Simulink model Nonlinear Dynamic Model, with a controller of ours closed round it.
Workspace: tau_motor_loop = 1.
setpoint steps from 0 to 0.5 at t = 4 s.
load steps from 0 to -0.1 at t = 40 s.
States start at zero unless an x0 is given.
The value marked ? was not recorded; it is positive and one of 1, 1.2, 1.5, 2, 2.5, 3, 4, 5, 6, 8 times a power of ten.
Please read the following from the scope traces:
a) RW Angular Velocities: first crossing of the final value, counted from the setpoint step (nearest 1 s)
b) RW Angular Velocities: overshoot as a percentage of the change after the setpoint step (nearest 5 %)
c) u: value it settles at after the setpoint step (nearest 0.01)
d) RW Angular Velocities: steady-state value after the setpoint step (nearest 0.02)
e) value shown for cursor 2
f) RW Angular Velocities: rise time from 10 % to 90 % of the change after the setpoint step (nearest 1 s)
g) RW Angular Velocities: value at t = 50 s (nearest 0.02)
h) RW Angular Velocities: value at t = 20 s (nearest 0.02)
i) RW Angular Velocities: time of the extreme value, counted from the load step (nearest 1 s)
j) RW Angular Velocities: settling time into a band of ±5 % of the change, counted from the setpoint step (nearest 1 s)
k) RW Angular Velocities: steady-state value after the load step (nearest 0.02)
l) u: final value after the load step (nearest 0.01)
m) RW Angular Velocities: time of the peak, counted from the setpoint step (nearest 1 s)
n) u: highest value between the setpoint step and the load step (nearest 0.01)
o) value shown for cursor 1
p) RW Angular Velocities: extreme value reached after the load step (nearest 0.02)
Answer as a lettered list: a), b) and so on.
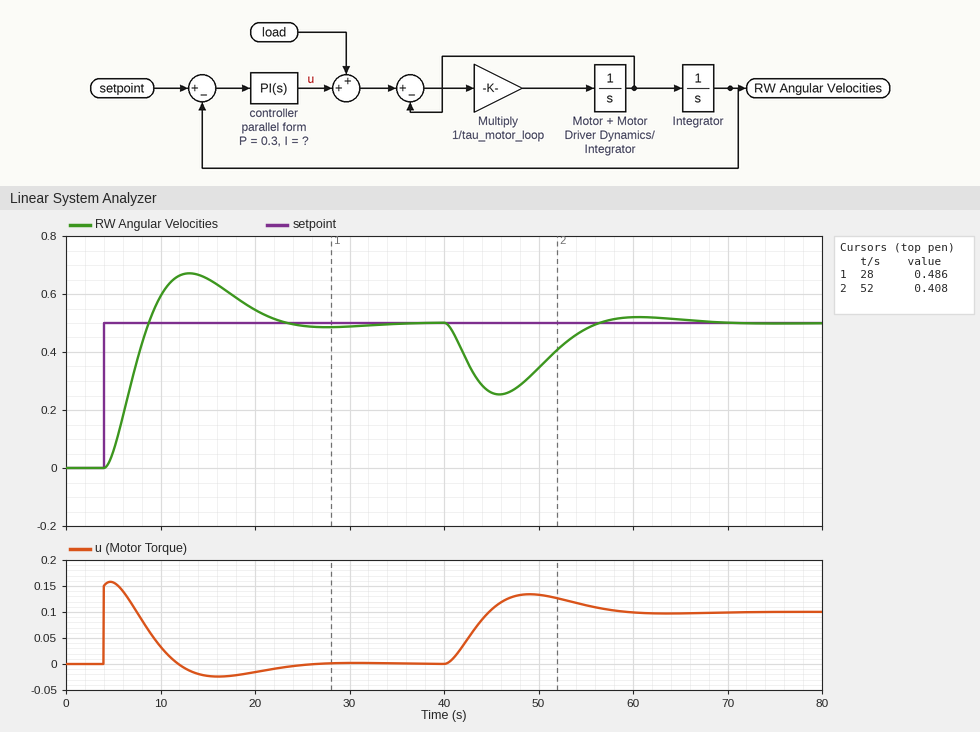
a) 5 s
b) 35 %
c) 0.00
d) 0.50
e) 0.408
f) 3 s
g) 0.34
h) 0.54
i) 6 s
j) 17 s
k) 0.50
l) 0.10
m) 9 s
n) 0.16
o) 0.486
p) 0.26
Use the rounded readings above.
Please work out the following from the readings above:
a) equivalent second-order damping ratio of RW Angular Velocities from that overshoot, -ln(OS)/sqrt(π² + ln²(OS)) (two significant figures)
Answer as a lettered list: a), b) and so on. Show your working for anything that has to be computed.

a) ln(0.35) = -1.050; 1.050 / sqrt(9.870 + 1.102) = 0.32
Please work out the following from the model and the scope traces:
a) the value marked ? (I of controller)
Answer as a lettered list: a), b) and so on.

a) 0.05
